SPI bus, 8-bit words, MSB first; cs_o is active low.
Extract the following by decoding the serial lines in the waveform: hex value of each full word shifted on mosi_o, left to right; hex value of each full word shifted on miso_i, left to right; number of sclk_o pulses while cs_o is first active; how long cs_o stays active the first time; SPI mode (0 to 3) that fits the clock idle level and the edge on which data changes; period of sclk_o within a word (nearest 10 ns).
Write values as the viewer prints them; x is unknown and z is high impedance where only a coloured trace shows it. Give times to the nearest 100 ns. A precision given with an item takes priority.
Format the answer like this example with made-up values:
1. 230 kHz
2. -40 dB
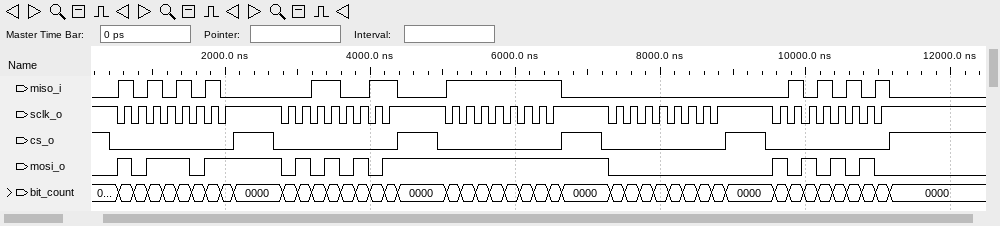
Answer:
1. BB, 55, FF, 00, AA
2. AA, 33, FF, 00, 55
3. 8
4. 1700 ns
5. 3
6. 200 ns
